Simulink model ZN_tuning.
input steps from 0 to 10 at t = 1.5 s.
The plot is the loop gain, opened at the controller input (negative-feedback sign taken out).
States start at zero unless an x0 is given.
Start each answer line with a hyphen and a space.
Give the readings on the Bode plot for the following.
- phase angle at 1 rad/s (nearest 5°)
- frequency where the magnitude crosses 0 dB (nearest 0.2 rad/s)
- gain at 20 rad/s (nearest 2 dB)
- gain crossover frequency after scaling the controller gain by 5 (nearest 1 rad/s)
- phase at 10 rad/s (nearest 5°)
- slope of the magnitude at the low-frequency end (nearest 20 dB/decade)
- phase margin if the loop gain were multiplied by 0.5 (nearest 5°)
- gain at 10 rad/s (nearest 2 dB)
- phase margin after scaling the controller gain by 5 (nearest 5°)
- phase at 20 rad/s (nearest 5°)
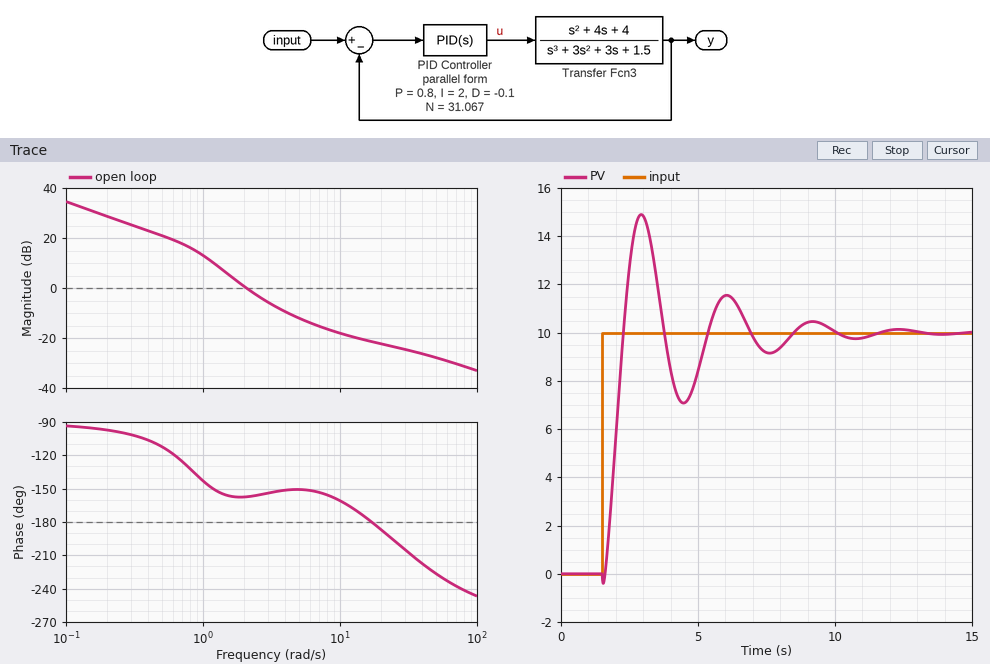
- -145°
- 2.0 rad/s
- -22 dB
- 6 rad/s
- -160°
- -20 dB/decade
- 25°
- -18 dB
- 30°
- -185°
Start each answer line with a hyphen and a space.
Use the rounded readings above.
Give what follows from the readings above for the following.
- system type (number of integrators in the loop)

- 1
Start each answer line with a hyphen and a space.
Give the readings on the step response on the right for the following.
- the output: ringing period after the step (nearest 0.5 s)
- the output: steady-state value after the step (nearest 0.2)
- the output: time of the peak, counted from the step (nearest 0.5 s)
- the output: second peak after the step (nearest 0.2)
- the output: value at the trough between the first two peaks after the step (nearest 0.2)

- 3.0 s
- 10.0
- 1.5 s
- 11.6
- 7.0
